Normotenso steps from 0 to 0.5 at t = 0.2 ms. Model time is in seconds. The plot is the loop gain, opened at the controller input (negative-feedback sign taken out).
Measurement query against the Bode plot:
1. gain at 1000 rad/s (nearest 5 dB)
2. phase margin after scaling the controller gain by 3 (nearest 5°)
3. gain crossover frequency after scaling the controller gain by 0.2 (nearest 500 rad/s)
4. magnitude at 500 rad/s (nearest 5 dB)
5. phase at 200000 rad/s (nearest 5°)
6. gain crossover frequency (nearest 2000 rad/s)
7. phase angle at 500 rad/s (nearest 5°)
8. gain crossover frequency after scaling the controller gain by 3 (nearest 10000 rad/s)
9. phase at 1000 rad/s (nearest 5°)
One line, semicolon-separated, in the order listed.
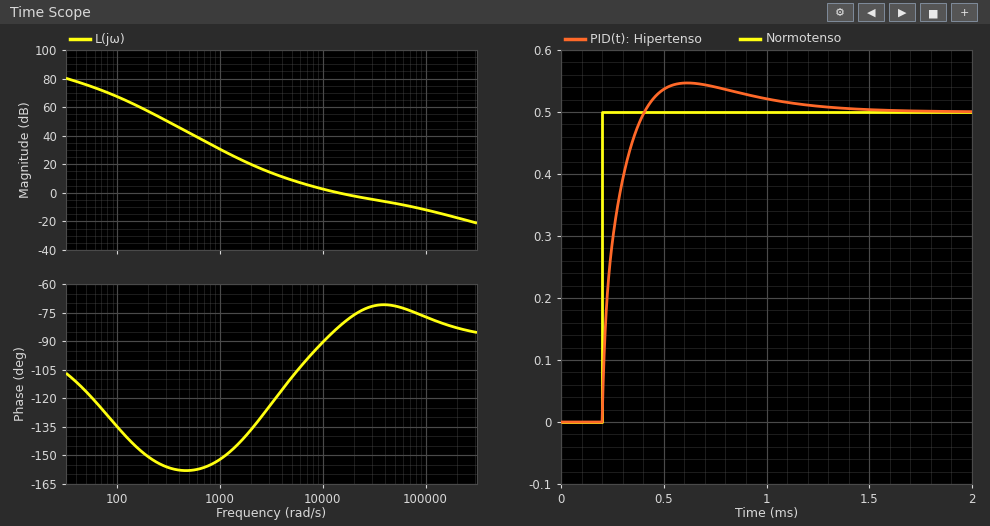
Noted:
30 dB; 105°; 3000 rad/s; 40 dB; -85°; 14000 rad/s; -160°; 70000 rad/s; -150°
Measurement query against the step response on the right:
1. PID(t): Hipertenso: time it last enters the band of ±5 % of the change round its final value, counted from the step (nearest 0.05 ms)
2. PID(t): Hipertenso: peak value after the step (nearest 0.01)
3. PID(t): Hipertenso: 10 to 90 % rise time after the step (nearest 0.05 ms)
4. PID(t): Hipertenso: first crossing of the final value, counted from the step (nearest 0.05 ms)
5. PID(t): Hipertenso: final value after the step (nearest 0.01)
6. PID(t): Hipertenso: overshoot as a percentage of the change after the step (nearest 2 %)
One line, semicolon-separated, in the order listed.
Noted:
0.75 ms; 0.55; 0.15 ms; 0.20 ms; 0.50; 10 %
